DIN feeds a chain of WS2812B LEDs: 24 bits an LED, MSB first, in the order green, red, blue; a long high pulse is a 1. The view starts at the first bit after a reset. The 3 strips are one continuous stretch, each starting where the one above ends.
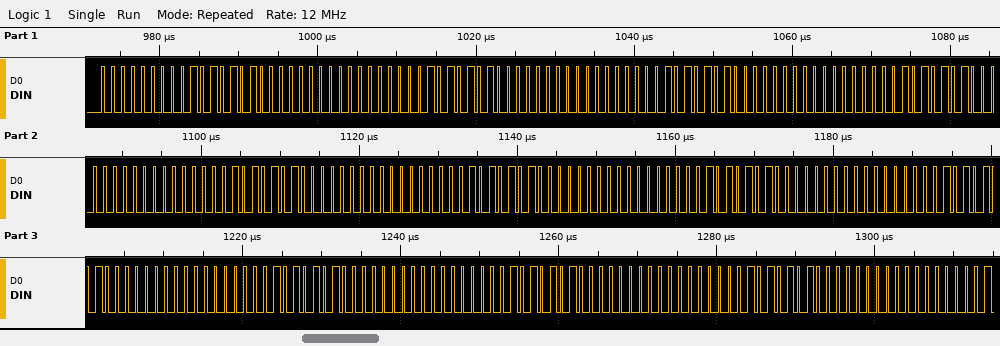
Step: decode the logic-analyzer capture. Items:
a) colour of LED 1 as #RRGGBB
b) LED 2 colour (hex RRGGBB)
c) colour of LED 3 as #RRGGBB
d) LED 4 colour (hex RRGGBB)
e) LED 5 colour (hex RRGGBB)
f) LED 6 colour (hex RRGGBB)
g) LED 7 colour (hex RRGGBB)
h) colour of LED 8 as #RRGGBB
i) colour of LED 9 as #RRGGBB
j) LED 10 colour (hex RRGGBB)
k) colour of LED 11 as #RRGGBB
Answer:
#550000
#550000
#550000
#550000
#550000
#550000
#550000
#550000
#550000
#550000
#550000
